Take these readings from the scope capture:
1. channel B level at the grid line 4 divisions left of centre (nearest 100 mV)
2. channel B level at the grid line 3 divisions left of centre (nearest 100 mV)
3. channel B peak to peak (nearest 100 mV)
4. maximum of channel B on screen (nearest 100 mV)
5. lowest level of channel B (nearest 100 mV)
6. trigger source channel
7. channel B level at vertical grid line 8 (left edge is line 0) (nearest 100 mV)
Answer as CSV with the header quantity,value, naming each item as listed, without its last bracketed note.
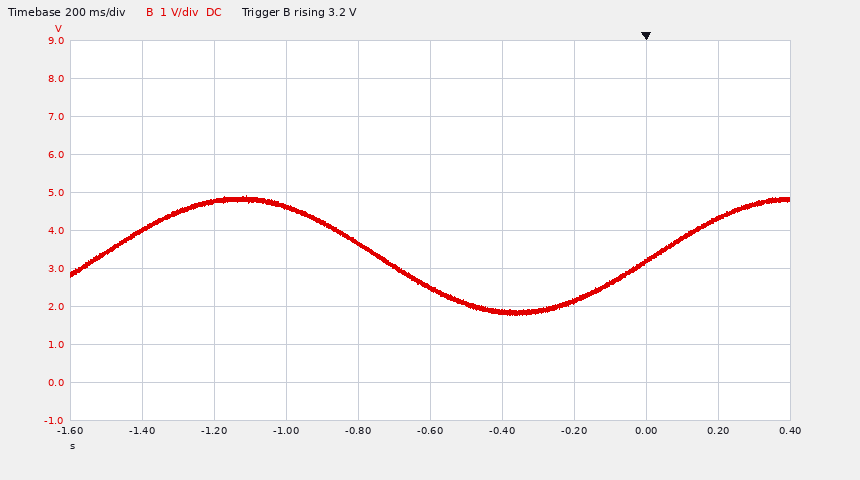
quantity,value
channel B level at the grid line 4 divisions left of centre,4.0 V
channel B level at the grid line 3 divisions left of centre,4.8 V
channel B peak to peak,3.1 V
maximum of channel B on screen,4.9 V
lowest level of channel B,1.8 V
trigger source channel,channel B
channel B level at vertical grid line 8 (left edge is line 0),3.2 V
